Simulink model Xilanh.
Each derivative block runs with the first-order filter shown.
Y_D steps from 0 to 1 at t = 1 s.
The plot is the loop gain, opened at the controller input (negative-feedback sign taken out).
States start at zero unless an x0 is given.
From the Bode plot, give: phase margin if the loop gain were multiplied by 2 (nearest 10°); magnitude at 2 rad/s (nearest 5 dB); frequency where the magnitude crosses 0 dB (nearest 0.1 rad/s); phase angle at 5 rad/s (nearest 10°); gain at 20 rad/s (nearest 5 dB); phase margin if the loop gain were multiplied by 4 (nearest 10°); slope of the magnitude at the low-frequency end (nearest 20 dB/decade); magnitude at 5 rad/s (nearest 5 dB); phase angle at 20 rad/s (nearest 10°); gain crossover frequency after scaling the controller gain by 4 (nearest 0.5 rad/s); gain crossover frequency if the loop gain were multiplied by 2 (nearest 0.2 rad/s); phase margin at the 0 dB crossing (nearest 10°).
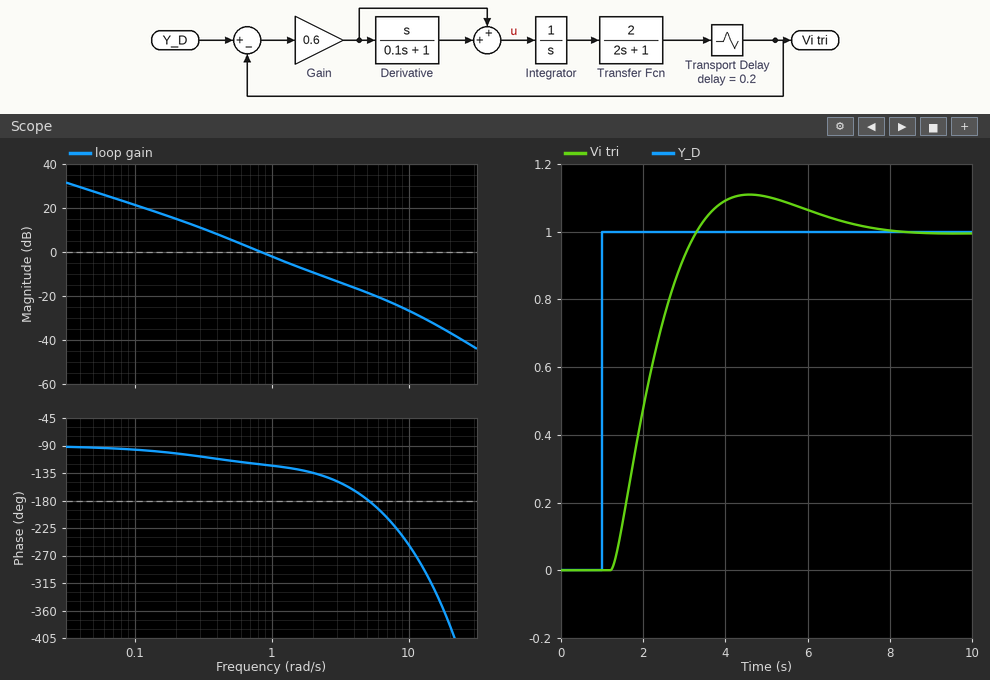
50°
-10 dB
0.8 rad/s
-180°
-35 dB
40°
-20 dB/decade
-20 dB
-380°
2.5 rad/s
1.4 rad/s
60°
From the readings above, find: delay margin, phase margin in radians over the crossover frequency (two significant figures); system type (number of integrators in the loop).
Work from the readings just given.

1.3 s
1
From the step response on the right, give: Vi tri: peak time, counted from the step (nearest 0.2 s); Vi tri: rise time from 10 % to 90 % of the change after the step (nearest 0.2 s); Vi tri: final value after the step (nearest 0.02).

3.6 s
1.4 s
1.00
